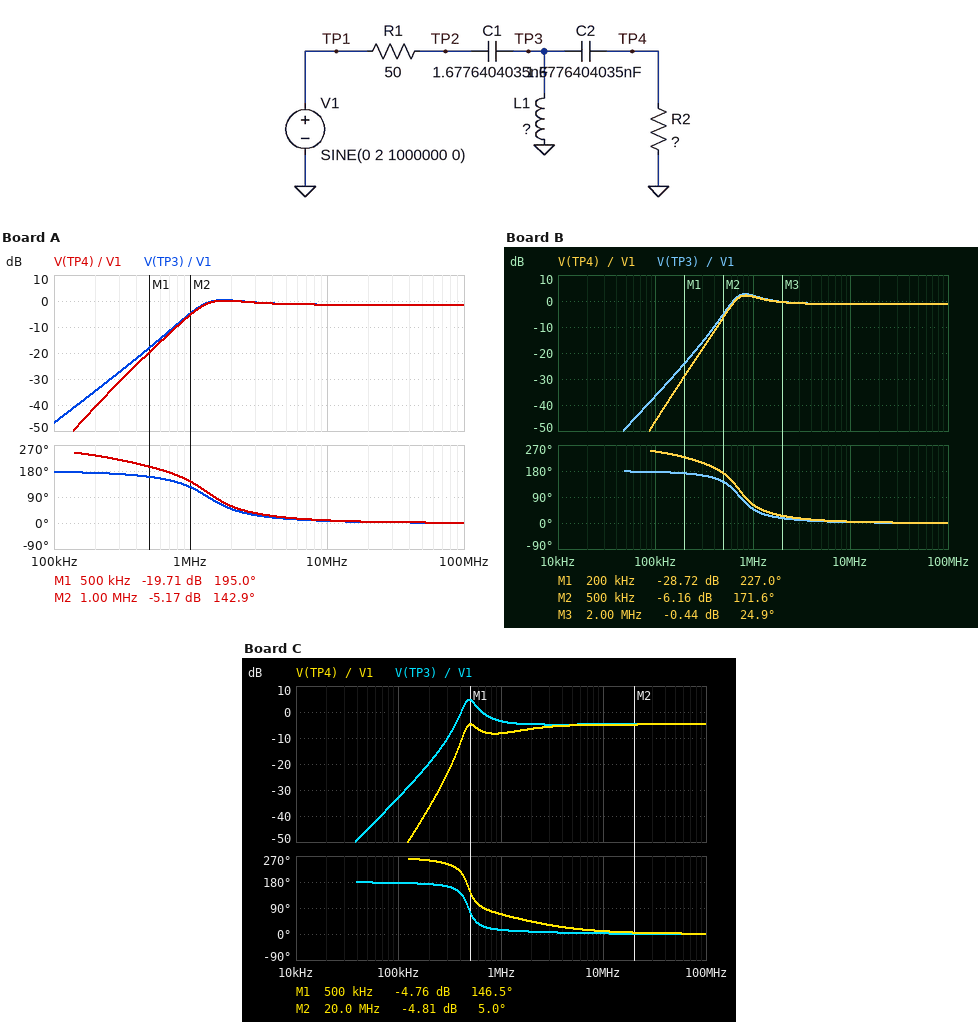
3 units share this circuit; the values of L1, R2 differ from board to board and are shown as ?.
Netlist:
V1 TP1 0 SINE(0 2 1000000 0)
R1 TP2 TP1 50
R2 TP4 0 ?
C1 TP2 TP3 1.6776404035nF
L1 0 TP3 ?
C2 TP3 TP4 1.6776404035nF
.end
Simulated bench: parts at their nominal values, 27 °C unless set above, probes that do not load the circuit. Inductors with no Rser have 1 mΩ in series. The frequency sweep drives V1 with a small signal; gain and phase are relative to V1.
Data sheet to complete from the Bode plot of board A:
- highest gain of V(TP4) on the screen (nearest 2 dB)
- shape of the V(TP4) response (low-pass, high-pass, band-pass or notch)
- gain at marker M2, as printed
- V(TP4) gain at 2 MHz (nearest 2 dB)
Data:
0 dB
high-pass
-5.17 dB
0 dB
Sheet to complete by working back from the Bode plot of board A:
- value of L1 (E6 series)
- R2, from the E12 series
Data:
6.8 µH
270 Ω
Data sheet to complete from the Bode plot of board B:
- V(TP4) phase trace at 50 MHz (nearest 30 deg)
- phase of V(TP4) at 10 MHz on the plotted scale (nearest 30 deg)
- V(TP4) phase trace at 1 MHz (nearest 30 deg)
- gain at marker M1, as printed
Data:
0 deg
0 deg
60 deg
-28.72 dB
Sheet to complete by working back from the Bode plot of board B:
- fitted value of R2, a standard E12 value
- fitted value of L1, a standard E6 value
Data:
330 Ω
22 µH
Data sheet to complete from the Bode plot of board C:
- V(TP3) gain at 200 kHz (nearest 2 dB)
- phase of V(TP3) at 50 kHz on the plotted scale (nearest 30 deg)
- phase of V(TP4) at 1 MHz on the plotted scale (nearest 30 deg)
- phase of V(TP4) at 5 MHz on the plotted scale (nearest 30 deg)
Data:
-20 dB
180 deg
60 deg
30 deg
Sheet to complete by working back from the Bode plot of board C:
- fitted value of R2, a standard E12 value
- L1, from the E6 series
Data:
68 Ω
33 µH
